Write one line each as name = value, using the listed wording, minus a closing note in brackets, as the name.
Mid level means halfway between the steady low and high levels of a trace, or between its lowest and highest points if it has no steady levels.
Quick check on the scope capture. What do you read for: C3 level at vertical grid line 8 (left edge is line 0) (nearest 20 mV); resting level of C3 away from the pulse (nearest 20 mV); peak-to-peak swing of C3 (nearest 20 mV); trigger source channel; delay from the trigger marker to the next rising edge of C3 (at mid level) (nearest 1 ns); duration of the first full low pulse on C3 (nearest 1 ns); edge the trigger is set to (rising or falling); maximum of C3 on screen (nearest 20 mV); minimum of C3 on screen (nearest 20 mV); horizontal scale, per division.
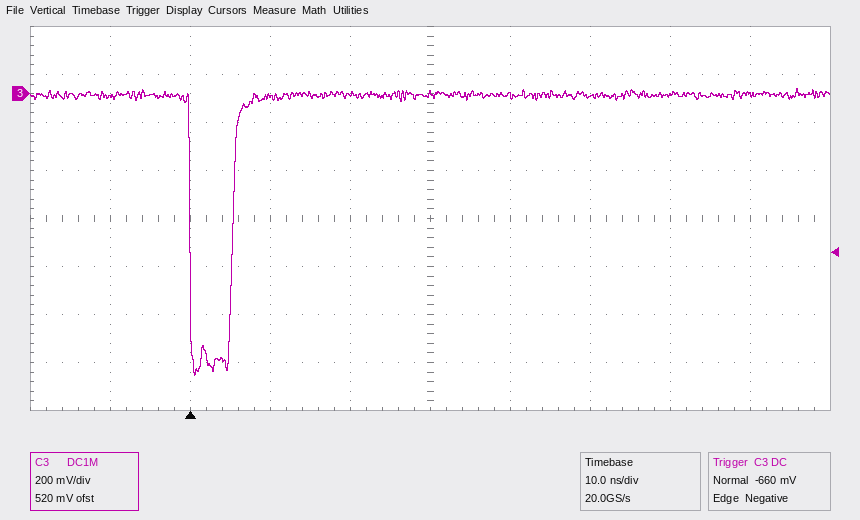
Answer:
C3 level at vertical grid line 8 (left edge is line 0) = 0 mV
resting level of C3 away from the pulse = 0 mV
peak-to-peak swing of C3 = 1.20 V
trigger source channel = C3
delay from the trigger marker to the next rising edge of C3 (at mid level) = 5 ns
duration of the first full low pulse on C3 = 5 ns
edge the trigger is set to = falling
maximum of C3 on screen = 20 mV
minimum of C3 on screen = -1.18 V
horizontal scale, per division = 10 ns
